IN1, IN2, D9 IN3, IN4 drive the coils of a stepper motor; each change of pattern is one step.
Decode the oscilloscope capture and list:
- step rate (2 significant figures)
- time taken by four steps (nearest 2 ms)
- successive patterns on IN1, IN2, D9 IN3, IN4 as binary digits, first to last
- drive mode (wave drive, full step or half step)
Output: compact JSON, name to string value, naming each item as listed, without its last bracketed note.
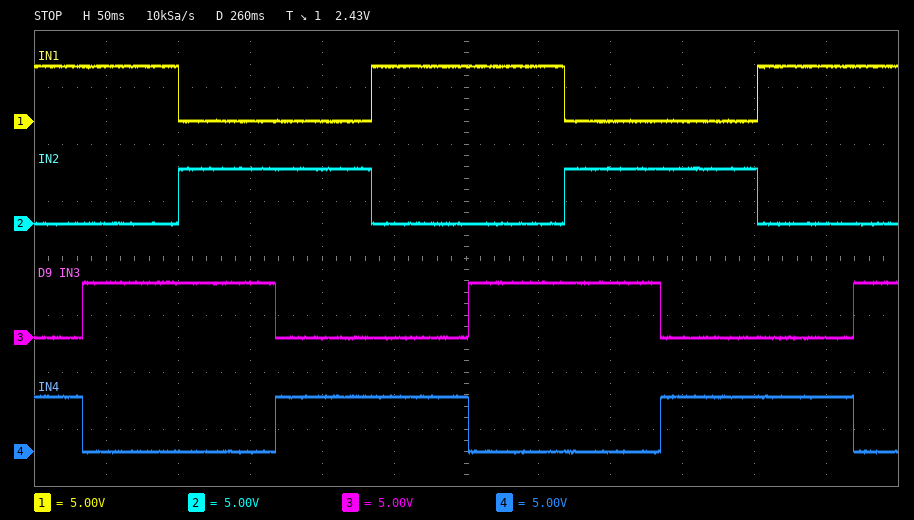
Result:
{"step rate": "15 steps/s", "time taken by four steps": "268 ms", "successive patterns on IN1, IN2, D9 IN3, IN4 as binary digits, first to last": "1001 1010 0110 0101 1001 1010 0110 0101 1001 1010", "drive mode": "full step"}
